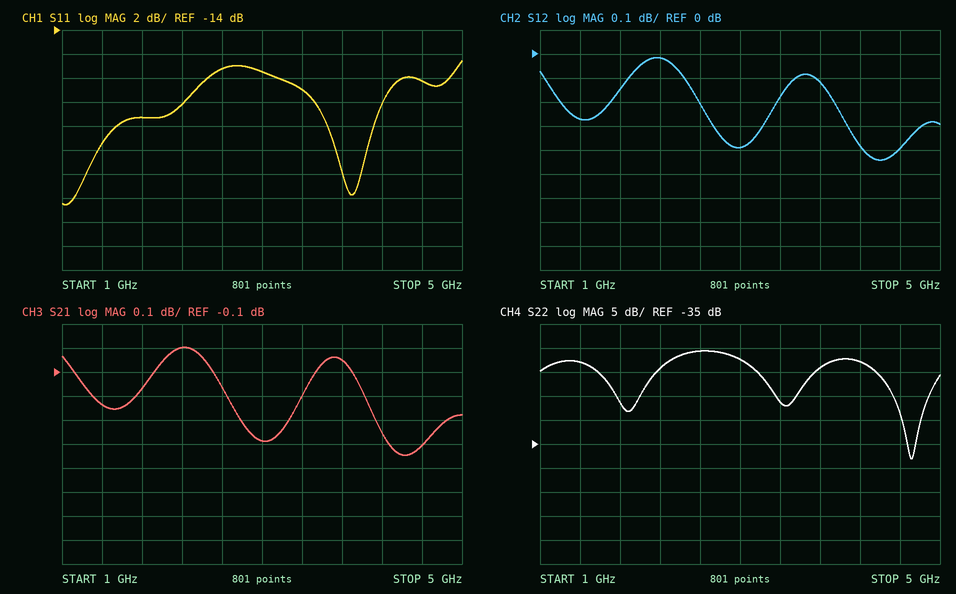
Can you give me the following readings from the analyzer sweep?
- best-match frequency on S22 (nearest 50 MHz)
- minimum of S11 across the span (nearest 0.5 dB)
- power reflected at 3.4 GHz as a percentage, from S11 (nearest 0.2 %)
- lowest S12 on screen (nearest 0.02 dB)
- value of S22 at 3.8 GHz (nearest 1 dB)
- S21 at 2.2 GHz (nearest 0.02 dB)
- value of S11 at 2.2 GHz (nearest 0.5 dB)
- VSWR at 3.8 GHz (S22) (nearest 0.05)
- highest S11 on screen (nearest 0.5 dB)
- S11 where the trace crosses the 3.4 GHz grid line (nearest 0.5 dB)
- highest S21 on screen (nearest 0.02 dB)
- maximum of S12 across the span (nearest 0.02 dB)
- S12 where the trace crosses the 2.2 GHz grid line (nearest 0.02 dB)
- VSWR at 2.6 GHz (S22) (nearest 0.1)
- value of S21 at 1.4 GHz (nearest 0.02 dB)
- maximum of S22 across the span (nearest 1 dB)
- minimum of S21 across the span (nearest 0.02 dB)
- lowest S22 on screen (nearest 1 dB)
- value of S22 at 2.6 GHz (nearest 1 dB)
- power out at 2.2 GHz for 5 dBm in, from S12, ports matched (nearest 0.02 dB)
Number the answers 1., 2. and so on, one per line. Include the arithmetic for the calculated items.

1. 4.70 GHz
2. -28.5 dB
3. 10^(-19/10) ≈ 1.26 %, so 1.2 % to the nearest 0.2 %
4. -0.44 dB
5. -19 dB
6. 0.00 dB
7. -20.0 dB
8. |Γ| = 10^(-19/20) = 0.1122; VSWR = (1 + 0.1122)/(1 − 0.1122) ≈ 1.25
9. -16.5 dB
10. -19.0 dB
11. 0.00 dB
12. -0.02 dB
13. -0.02 dB
14. |Γ| = 10^(-16/20) = 0.1585; VSWR = (1 + 0.1585)/(1 − 0.1585) ≈ 1.4
15. -0.24 dB
16. -16 dB
17. -0.44 dB
18. -38 dB
19. -16 dB
20. 5 dBm + (-0.02 dB) = 4.98 dBm
